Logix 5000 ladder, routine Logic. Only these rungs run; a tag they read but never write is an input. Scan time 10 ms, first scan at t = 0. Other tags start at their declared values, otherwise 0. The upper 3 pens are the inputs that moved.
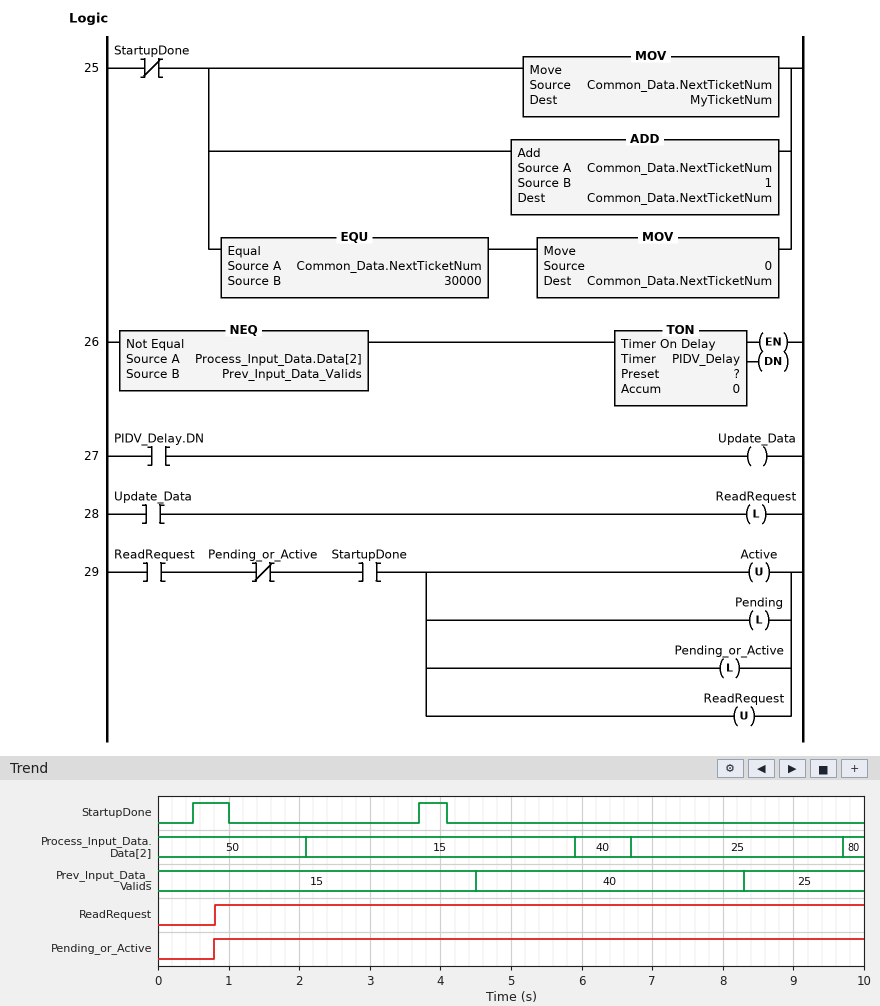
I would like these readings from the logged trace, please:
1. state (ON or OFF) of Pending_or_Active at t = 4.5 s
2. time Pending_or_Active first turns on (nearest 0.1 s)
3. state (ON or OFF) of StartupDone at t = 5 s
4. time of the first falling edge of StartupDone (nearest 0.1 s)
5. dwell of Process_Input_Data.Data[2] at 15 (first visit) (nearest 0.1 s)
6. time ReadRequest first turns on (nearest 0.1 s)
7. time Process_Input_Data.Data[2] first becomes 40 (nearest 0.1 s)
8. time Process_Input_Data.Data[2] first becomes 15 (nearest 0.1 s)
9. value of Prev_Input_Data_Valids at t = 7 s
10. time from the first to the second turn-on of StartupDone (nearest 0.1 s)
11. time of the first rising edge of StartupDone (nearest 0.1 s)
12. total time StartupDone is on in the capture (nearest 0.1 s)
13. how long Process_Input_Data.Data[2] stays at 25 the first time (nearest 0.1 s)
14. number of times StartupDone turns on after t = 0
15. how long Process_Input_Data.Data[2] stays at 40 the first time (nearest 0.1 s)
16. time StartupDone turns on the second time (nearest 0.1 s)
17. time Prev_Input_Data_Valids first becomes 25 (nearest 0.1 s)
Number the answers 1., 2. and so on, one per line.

1. ON
2. 0.8 s
3. OFF
4. 1.0 s
5. 3.8 s
6. 0.8 s
7. 5.9 s
8. 2.1 s
9. 40
10. 3.2 s
11. 0.5 s
12. 0.9 s
13. 3.0 s
14. 2
15. 0.8 s
16. 3.7 s
17. 8.3 s
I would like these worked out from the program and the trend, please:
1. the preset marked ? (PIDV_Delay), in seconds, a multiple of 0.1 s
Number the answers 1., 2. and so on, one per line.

1. 0.8 s
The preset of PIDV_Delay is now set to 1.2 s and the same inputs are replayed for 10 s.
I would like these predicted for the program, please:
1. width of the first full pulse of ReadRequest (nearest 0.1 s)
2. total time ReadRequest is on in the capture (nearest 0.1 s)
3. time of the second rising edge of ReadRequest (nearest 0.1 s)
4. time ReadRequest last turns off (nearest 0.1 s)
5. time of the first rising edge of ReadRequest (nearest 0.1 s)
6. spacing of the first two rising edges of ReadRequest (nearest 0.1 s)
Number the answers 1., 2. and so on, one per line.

1. 2.5 s
2. 6.8 s
3. 5.7 s
4. 3.7 s
5. 1.2 s
6. 4.5 s
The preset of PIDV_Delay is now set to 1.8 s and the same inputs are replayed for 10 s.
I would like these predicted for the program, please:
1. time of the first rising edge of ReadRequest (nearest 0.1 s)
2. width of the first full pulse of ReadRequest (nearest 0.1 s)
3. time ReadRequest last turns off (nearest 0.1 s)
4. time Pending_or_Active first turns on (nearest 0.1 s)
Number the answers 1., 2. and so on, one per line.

1. 1.8 s
2. 1.9 s
3. 3.7 s
4. 3.7 s
